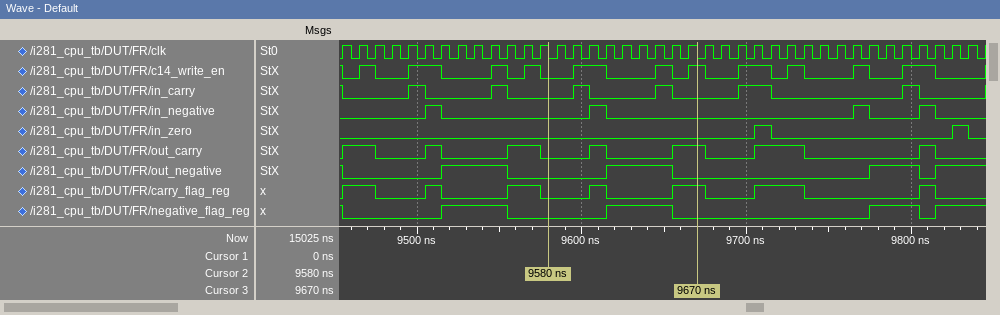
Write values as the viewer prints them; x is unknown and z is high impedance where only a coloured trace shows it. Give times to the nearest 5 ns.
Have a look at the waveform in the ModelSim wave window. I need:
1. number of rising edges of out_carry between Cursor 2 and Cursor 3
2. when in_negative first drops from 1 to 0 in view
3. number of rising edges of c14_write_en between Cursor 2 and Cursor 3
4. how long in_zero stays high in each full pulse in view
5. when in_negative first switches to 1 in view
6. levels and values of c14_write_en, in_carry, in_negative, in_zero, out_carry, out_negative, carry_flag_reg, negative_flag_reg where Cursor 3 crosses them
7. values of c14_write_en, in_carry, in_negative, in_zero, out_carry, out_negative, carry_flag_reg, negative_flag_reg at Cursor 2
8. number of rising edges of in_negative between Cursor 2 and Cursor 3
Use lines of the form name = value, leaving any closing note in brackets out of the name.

number of rising edges of out_carry between Cursor 2 and Cursor 3 = 2
when in_negative first drops from 1 to 0 in view = 9515 ns
number of rising edges of c14_write_en between Cursor 2 and Cursor 3 = 3
how long in_zero stays high in each full pulse in view = 10 ns, 10 ns
when in_negative first switches to 1 in view = 9505 ns
levels and values of c14_write_en, in_carry, in_negative, in_zero, out_carry, out_negative, carry_flag_reg, negative_flag_reg where Cursor 3 crosses them = c14_write_en=1, in_carry=0, in_negative=0, in_zero=0, out_carry=1, out_negative=0, carry_flag_reg=1, negative_flag_reg=0
values of c14_write_en, in_carry, in_negative, in_zero, out_carry, out_negative, carry_flag_reg, negative_flag_reg at Cursor 2 = c14_write_en=0, in_carry=0, in_negative=0, in_zero=0, out_carry=0, out_negative=0, carry_flag_reg=0, negative_flag_reg=0
number of rising edges of in_negative between Cursor 2 and Cursor 3 = 1
